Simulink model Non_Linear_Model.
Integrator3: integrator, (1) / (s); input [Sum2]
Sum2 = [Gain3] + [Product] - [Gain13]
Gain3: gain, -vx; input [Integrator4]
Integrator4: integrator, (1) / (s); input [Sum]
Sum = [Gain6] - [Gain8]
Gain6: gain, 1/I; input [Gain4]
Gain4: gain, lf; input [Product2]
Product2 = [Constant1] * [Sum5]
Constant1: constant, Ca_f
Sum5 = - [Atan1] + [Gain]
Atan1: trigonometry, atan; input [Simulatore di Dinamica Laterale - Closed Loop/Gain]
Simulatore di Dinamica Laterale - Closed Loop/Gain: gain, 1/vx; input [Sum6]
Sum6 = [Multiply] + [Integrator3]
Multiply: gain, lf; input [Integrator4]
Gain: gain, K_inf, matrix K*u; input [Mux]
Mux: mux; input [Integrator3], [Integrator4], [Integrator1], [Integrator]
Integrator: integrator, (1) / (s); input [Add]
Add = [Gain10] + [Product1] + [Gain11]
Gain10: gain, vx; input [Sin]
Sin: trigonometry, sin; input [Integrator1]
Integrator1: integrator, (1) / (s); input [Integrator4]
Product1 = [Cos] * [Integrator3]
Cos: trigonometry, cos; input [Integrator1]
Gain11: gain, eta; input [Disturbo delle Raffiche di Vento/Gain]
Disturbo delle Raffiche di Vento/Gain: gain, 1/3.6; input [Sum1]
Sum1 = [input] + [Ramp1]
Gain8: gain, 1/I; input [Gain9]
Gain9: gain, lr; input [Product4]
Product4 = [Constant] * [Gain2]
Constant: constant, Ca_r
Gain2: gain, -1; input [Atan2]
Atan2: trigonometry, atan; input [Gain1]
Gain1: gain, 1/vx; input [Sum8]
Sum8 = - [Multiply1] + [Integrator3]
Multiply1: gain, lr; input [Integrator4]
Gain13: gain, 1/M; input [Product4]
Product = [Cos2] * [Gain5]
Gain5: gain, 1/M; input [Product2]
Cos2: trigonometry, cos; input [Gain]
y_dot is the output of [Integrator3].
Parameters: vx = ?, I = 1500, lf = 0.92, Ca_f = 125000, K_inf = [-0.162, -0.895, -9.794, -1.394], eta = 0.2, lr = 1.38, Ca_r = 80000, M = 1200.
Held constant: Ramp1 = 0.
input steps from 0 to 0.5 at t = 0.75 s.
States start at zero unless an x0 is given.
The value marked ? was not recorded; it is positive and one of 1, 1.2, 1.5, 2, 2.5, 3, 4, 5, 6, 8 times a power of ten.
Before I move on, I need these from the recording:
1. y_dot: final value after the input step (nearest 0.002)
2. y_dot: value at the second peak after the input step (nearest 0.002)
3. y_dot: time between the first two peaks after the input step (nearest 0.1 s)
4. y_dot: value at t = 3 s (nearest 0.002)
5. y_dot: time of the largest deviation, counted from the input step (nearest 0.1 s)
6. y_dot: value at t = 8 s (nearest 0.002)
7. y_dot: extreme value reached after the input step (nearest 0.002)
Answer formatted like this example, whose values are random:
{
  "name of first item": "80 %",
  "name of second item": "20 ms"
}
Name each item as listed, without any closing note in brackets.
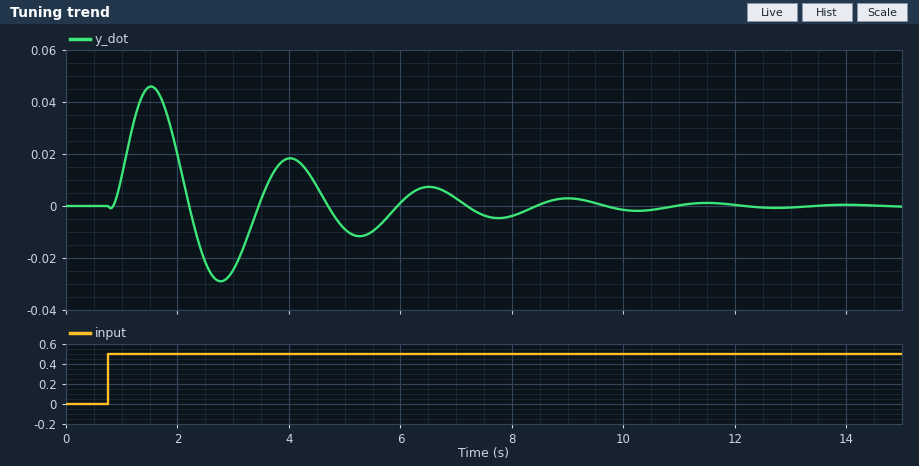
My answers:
{
  "y_dot: final value after the input step": "0.000",
  "y_dot: value at the second peak after the input step": "0.018",
  "y_dot: time between the first two peaks after the input step": "2.5 s",
  "y_dot: value at t = 3 s": "-0.024",
  "y_dot: time of the largest deviation, counted from the input step": "0.8 s",
  "y_dot: value at t = 8 s": "-0.004",
  "y_dot: extreme value reached after the input step": "0.046"
}
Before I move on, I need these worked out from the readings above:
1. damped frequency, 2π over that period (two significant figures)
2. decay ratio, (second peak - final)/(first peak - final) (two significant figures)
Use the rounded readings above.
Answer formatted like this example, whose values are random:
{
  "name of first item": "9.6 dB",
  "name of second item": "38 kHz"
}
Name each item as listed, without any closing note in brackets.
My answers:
{
  "damped frequency, 2π over that period": "2.5 rad/s",
  "decay ratio, (second peak - final)/(first peak - final)": "0.39"
}
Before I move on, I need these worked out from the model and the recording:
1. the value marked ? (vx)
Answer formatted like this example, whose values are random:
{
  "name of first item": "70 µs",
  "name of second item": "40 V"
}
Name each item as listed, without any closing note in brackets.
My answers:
{
  "the value marked ?": "30"
}
